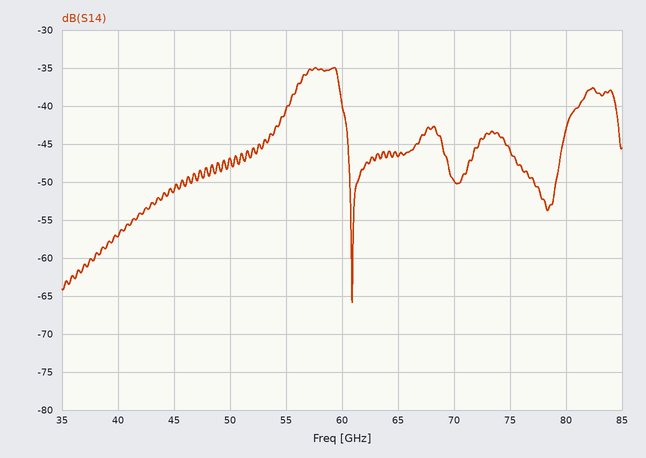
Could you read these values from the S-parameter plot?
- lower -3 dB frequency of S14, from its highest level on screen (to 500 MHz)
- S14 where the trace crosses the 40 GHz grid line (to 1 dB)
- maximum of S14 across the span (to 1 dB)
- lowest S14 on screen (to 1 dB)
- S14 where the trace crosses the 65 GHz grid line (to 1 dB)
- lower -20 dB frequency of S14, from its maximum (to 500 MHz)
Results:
56.0 GHz
-57 dB
-35 dB
-66 dB
-47 dB
41.5 GHz
